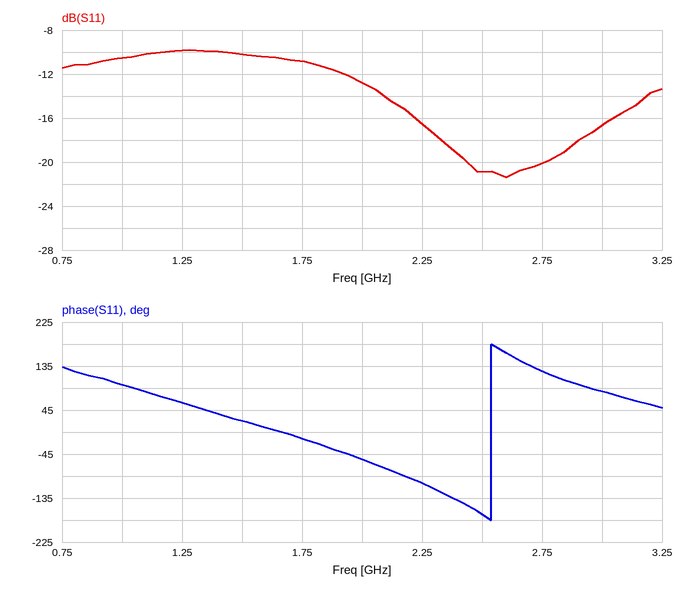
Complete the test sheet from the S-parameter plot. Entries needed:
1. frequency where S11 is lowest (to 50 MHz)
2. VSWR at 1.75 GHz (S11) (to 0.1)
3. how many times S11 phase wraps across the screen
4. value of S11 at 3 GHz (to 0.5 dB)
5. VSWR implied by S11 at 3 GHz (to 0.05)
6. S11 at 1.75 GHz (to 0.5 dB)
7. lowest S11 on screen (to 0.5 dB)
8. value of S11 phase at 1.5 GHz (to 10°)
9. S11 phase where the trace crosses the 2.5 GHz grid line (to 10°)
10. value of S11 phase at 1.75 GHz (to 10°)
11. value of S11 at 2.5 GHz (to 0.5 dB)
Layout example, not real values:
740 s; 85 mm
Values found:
2.60 GHz; 1.8; 1; -16.5 dB; 1.35; -11.0 dB; -21.5 dB; 20°; -170°; -10°; -21.0 dB
